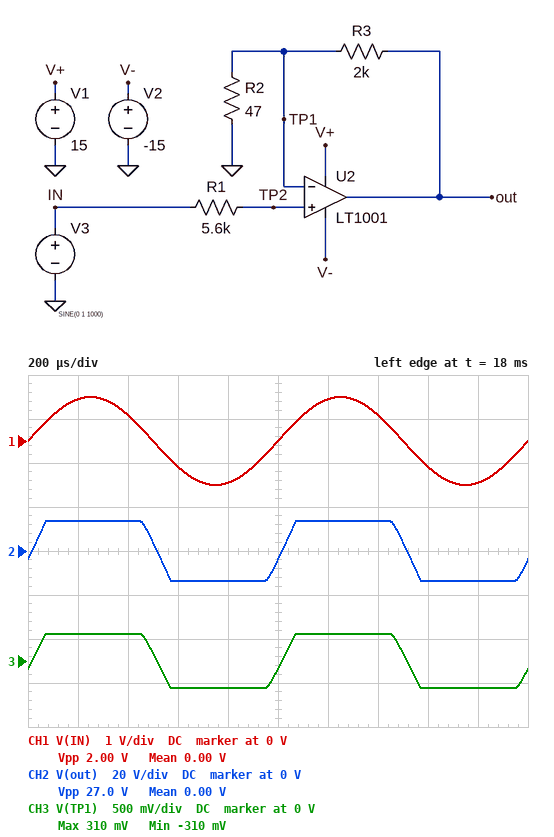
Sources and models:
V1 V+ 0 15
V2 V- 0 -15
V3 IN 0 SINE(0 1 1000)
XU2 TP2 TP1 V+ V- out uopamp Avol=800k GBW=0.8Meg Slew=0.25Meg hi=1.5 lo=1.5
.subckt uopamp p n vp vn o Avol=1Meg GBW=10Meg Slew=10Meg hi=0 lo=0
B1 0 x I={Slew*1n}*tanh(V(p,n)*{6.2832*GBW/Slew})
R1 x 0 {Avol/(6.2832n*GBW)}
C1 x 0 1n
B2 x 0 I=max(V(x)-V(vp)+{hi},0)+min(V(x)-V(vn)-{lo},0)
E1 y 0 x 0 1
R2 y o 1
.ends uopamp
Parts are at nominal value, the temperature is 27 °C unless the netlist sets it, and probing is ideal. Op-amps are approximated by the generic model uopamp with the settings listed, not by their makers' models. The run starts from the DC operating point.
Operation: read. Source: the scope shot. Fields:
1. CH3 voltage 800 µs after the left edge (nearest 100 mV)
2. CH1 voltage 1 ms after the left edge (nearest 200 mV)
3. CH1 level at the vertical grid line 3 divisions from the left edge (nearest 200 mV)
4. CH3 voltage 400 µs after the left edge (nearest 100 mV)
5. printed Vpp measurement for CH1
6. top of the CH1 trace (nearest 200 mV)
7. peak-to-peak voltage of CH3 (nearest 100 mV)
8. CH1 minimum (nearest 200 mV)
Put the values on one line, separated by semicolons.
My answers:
-300 mV; 0 V; -600 mV; 300 mV; 2.00 V; 1.0 V; 600 mV; -1.0 V
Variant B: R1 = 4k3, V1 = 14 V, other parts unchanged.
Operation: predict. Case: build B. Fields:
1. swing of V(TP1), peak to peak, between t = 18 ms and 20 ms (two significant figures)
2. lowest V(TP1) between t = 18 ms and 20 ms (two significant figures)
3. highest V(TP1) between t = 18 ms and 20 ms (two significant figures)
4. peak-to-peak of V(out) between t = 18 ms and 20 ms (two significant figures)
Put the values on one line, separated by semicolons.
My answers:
600 mV; -310 mV; 290 mV; 26 V
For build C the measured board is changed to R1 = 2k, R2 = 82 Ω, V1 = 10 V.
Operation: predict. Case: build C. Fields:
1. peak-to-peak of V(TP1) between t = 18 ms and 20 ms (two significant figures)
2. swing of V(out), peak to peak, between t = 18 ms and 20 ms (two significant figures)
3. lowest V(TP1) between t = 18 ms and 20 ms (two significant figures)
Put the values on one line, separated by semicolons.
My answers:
870 mV; 22 V; -530 mV
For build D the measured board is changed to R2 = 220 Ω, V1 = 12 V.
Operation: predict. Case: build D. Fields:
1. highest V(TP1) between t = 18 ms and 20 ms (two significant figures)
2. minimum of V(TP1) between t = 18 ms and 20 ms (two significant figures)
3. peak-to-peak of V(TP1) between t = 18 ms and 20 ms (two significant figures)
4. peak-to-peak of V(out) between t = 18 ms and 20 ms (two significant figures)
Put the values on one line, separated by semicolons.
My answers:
1.0 V; -1.0 V; 2.0 V; 20 V
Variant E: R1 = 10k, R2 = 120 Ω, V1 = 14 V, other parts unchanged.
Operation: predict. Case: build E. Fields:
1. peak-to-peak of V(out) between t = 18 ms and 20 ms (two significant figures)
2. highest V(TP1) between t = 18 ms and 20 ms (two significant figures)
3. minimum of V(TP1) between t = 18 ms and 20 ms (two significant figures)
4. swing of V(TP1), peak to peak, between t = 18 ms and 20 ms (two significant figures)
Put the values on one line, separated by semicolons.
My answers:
26 V; 710 mV; -760 mV; 1.5 V
